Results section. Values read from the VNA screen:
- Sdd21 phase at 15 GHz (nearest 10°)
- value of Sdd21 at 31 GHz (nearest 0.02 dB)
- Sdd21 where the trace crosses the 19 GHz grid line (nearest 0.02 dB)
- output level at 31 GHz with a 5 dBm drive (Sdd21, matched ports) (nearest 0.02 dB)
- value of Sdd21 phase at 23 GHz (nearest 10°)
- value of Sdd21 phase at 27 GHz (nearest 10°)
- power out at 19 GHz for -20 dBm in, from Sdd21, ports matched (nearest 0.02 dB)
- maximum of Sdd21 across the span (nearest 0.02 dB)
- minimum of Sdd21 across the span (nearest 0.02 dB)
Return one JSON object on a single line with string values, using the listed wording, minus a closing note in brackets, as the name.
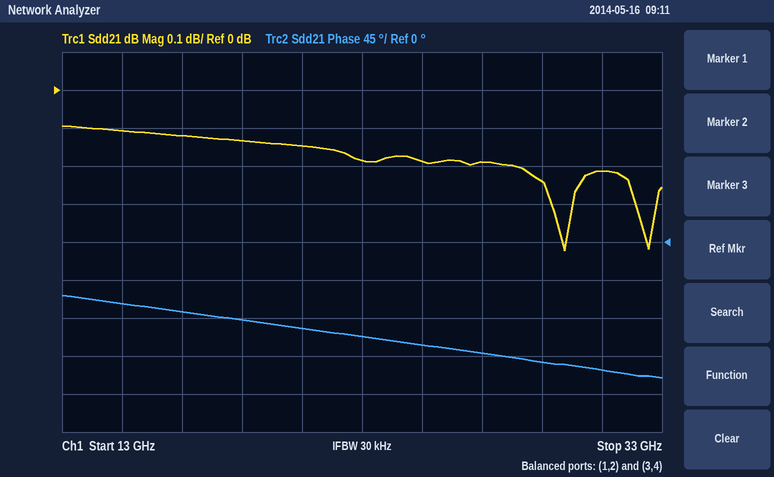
{"Sdd21 phase at 15 GHz": "-70°", "value of Sdd21 at 31 GHz": "-0.22 dB", "Sdd21 where the trace crosses the 19 GHz grid line": "-0.14 dB", "output level at 31 GHz with a 5 dBm drive (Sdd21, matched ports)": "4.78 dBm", "value of Sdd21 phase at 23 GHz": "-110°", "value of Sdd21 phase at 27 GHz": "-130°", "power out at 19 GHz for -20 dBm in, from Sdd21, ports matched": "-20.14 dBm", "maximum of Sdd21 across the span": "-0.10 dB", "minimum of Sdd21 across the span": "-0.42 dB"}
